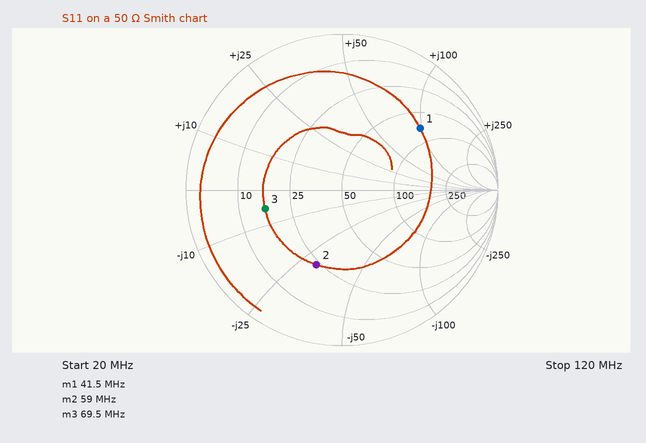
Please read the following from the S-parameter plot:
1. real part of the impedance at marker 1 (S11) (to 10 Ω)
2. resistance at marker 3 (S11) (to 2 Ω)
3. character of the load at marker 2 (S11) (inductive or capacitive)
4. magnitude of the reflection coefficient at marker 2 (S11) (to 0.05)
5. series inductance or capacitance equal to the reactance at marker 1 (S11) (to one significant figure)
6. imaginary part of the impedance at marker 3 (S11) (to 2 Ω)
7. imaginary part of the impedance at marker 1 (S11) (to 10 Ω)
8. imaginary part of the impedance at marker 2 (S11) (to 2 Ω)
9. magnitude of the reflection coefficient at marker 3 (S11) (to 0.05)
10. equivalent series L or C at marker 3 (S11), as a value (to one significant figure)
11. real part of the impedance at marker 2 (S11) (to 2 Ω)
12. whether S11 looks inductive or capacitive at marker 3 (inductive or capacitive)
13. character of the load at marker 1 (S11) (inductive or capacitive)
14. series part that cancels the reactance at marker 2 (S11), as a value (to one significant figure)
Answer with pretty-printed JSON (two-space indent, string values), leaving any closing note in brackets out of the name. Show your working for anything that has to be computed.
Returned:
{
  "real part of the impedance at marker 1 (S11)": "70 Ω",
  "resistance at marker 3 (S11)": "16 Ω",
  "character of the load at marker 2 (S11)": "capacitive",
  "magnitude of the reflection coefficient at marker 2 (S11)": "0.50",
  "series inductance or capacitance equal to the reactance at marker 1 (S11)": "L = 100 Ω/(2π × 41.5 MHz) ≈ 384 nH, so 400 nH to one significant figure",
  "imaginary part of the impedance at marker 3 (S11)": "-6 Ω",
  "imaginary part of the impedance at marker 1 (S11)": "+100 Ω",
  "imaginary part of the impedance at marker 2 (S11)": "-30 Ω",
  "magnitude of the reflection coefficient at marker 3 (S11)": "0.50",
  "equivalent series L or C at marker 3 (S11), as a value": "C = 1/(2π × 69.5 MHz × 6 Ω) ≈ 382 pF, so 400 pF to one significant figure",
  "real part of the impedance at marker 2 (S11)": "24 Ω",
  "whether S11 looks inductive or capacitive at marker 3": "capacitive",
  "character of the load at marker 1 (S11)": "inductive",
  "series part that cancels the reactance at marker 2 (S11), as a value": "L = 30 Ω/(2π × 59 MHz) ≈ 80.9 nH, so 80 nH to one significant figure"
}
